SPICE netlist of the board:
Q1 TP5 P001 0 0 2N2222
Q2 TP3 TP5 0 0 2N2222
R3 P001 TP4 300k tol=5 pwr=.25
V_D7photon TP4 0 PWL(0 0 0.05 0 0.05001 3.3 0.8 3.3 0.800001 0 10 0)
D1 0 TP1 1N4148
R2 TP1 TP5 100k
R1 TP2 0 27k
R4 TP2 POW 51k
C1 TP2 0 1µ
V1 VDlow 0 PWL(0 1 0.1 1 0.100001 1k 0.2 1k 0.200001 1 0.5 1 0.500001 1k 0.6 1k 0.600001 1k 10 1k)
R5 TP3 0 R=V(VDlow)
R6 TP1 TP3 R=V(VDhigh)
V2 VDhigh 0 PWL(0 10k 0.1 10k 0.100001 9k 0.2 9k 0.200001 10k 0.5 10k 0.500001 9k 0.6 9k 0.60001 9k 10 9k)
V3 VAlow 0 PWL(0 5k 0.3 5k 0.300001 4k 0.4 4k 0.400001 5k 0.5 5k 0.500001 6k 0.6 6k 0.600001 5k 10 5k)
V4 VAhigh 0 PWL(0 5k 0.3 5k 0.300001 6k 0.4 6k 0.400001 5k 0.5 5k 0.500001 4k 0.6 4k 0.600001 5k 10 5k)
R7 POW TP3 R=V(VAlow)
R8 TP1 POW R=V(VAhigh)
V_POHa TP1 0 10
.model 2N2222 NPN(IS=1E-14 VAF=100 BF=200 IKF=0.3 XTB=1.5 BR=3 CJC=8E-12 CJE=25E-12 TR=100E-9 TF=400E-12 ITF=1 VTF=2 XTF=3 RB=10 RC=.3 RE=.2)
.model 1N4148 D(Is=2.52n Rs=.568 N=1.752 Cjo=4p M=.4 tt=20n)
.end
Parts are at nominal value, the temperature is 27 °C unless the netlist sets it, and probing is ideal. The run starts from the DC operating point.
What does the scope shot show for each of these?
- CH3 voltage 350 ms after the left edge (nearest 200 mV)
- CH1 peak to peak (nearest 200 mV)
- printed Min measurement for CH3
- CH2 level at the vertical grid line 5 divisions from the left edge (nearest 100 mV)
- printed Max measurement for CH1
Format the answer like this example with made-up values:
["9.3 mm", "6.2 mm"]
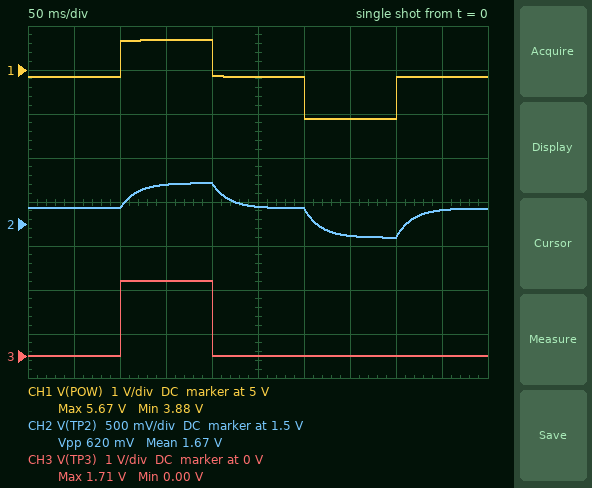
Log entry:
["0 V", "1.8 V", "0.00 V", "1.7 V", "5.67 V"]
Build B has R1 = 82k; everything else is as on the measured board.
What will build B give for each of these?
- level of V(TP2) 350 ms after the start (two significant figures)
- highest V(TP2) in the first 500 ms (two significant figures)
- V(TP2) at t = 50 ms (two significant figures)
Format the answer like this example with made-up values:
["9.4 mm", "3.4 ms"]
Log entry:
["2.6 V", "3.5 V", "3.0 V"]
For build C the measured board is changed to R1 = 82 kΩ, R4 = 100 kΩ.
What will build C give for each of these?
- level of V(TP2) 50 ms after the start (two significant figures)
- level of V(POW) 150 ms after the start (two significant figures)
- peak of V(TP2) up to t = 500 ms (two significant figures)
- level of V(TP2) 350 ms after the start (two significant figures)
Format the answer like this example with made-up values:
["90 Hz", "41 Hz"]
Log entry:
["2.2 V", "5.8 V", "2.6 V", "1.9 V"]
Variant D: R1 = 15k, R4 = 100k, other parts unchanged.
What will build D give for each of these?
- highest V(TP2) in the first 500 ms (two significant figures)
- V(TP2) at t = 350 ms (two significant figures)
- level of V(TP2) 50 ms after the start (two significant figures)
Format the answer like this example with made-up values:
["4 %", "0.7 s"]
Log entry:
["750 mV", "510 mV", "640 mV"]
